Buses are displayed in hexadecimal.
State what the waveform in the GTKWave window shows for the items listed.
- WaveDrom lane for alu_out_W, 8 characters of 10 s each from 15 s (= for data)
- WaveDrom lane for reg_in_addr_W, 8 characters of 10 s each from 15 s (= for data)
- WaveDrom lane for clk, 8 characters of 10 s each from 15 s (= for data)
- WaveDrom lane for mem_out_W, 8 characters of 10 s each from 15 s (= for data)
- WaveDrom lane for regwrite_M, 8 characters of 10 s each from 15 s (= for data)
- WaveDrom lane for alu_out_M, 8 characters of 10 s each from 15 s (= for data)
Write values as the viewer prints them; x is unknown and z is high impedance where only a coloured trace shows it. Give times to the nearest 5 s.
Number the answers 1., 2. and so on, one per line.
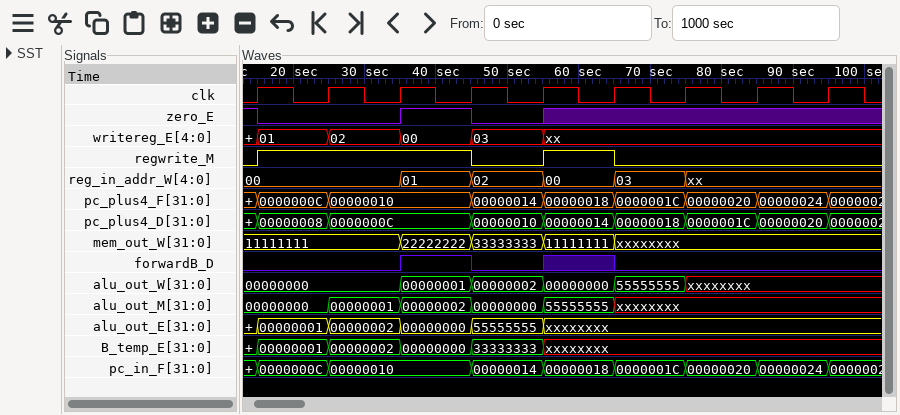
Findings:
1. {name: 'alu_out_W', wave: '=.====x.', data: '00000000 00000001 00000002 00000000 55555555'}
2. {name: 'reg_in_addr_W', wave: '=.====x.', data: '00 01 02 00 03'}
3. {name: 'clk', wave: 'p.......'}
4. {name: 'mem_out_W', wave: '=.===x..', data: '11111111 22222222 33333333 11111111'}
5. {name: 'regwrite_M', wave: '1..010..'}
6. {name: 'alu_out_M', wave: '=====x..', data: '00000000 00000001 00000002 00000000 55555555'}
